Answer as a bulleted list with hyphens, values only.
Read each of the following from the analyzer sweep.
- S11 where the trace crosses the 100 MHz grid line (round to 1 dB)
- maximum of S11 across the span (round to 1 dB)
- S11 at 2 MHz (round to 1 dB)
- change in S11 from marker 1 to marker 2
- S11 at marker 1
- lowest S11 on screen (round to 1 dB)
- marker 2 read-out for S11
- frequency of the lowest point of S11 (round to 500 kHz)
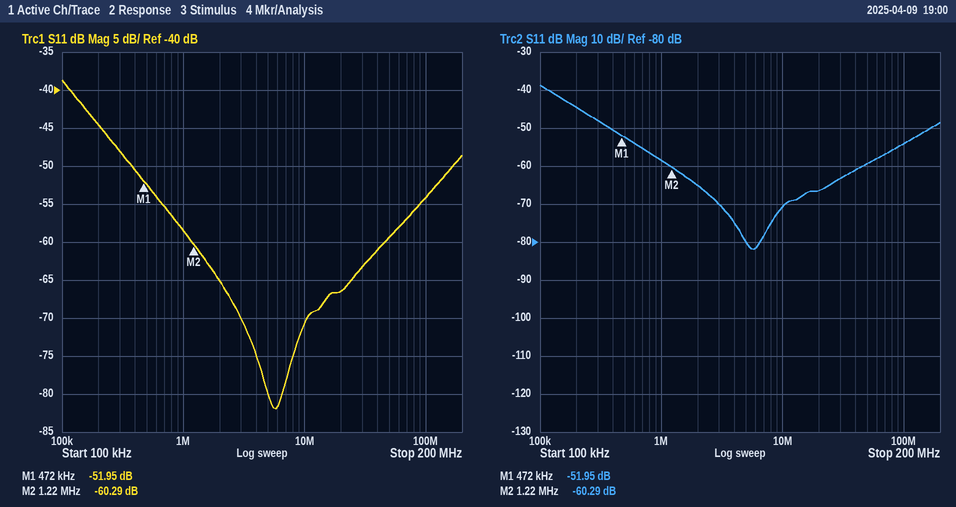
- -54 dB
- -39 dB
- -65 dB
- -8.34 dB
- -51.95 dB
- -82 dB
- -60.29 dB
- 6.0 MHz
